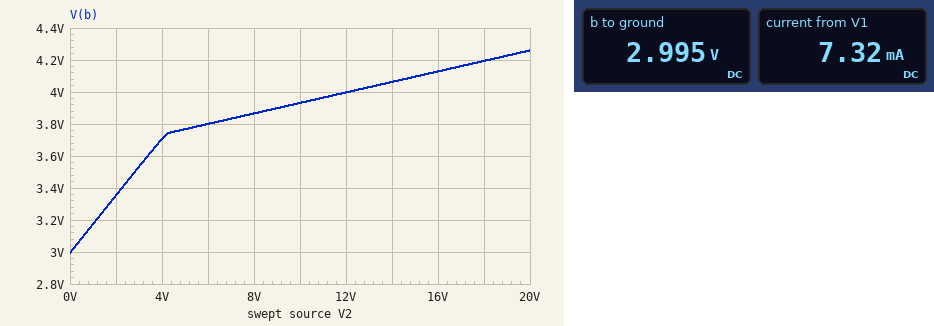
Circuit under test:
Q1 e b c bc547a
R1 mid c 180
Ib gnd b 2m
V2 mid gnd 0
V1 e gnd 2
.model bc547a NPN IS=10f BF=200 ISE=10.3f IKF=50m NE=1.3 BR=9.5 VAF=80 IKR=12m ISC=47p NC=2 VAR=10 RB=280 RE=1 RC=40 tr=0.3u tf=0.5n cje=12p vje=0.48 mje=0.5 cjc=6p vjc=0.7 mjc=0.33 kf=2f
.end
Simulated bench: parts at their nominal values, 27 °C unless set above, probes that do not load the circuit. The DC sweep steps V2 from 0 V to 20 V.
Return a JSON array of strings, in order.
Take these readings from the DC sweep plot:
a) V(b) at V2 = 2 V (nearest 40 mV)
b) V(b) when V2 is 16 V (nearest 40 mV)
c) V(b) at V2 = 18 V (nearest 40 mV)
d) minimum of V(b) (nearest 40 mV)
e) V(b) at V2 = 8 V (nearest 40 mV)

["3.36 V", "4.12 V", "4.20 V", "3.00 V", "3.88 V"]
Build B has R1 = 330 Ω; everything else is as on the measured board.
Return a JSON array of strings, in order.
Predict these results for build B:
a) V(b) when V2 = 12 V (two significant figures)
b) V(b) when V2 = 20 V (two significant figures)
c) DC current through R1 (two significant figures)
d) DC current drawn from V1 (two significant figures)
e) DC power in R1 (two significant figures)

["3.9 V", "4.2 V", "5.6 mA", "3.6 mA", "10 mW"]
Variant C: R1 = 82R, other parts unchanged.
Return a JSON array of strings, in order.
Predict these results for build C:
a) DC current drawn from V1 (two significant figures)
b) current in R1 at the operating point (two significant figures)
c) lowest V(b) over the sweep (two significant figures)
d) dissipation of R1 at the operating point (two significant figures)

["15 mA", "17 mA", "2.7 V", "23 mW"]
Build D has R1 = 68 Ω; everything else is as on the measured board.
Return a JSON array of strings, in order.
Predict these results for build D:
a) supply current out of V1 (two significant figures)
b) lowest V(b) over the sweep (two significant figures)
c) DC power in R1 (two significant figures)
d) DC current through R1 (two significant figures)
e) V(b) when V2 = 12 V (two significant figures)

["17 mA", "2.6 V", "24 mW", "19 mA", "4.1 V"]
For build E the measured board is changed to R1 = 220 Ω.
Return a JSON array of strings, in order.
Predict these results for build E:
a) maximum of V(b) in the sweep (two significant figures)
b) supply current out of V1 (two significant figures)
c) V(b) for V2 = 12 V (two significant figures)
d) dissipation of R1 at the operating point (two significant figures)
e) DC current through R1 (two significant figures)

["4.2 V", "5.9 mA", "4.0 V", "14 mW", "7.9 mA"]
